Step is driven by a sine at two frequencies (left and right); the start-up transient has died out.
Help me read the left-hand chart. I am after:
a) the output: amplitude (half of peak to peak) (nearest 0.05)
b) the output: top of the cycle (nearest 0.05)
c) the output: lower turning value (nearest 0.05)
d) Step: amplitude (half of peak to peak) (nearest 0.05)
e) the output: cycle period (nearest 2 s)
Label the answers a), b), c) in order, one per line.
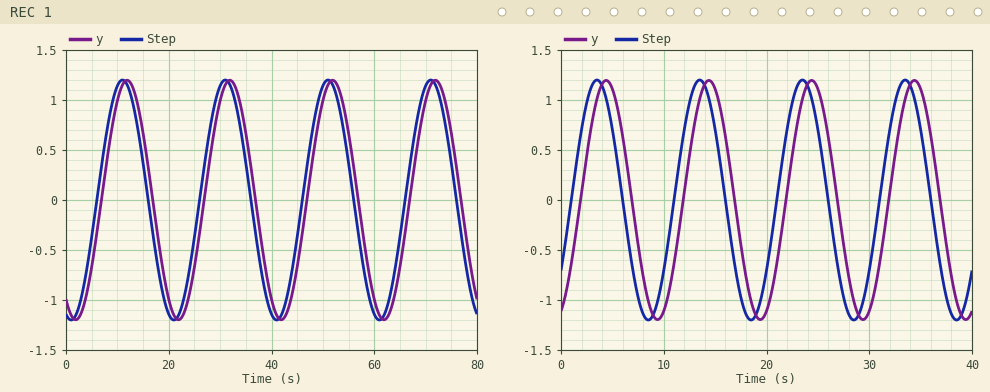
a) 1.20
b) 1.20
c) -1.20
d) 1.20
e) 20 s
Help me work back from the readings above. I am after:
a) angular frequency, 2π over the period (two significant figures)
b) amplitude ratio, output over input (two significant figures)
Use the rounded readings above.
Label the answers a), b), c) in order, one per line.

a) 0.31 rad/s
b) 1.0
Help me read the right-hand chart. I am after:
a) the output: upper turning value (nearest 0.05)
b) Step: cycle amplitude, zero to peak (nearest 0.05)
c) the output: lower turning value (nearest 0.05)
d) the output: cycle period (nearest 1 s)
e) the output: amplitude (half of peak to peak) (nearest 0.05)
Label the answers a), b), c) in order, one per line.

a) 1.20
b) 1.20
c) -1.20
d) 10 s
e) 1.20
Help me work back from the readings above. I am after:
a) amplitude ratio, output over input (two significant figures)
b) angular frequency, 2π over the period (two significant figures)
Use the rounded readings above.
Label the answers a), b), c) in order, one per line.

a) 1.0
b) 0.63 rad/s
